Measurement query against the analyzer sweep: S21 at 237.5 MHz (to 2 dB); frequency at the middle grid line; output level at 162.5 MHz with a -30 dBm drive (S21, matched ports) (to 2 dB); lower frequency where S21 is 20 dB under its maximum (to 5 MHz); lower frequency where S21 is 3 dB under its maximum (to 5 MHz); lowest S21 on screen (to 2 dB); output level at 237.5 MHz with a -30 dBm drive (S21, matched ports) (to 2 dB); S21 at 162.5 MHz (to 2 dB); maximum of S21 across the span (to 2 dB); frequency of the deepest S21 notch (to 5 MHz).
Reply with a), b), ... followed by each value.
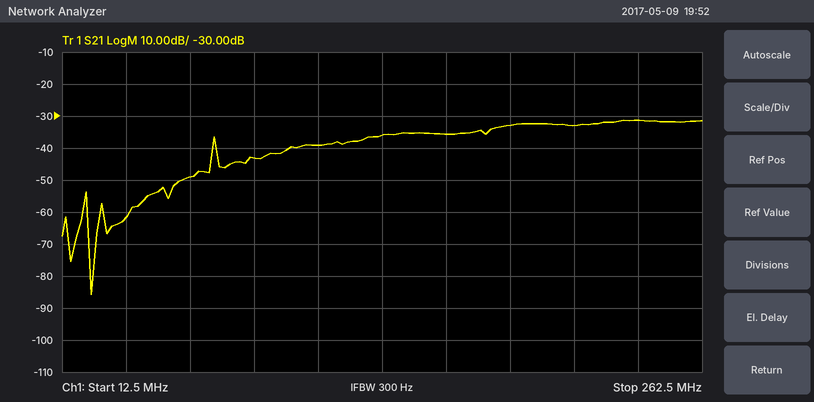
a) -32 dB
b) 137.5 MHz
c) -66 dBm
d) 55 MHz
e) 180 MHz
f) -86 dB
g) -62 dBm
h) -36 dB
i) -32 dB
j) 25 MHz
